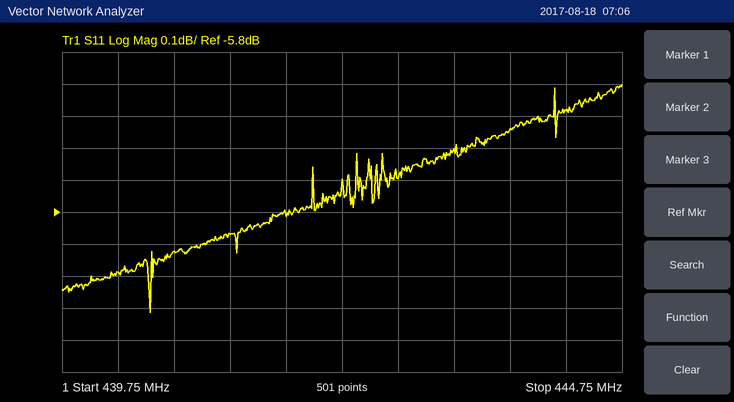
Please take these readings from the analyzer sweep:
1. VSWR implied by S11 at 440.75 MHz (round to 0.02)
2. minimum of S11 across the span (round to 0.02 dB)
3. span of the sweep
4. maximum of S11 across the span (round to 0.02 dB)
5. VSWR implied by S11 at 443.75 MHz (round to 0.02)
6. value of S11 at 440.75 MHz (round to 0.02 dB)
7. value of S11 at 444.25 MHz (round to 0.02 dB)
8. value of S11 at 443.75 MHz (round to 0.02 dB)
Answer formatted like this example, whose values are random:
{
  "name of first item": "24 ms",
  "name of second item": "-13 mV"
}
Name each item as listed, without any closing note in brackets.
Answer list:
{
  "VSWR implied by S11 at 440.75 MHz": "3.04",
  "minimum of S11 across the span": "-6.12 dB",
  "span of the sweep": "5 MHz",
  "maximum of S11 across the span": "-5.40 dB",
  "VSWR implied by S11 at 443.75 MHz": "3.24",
  "value of S11 at 440.75 MHz": "-5.92 dB",
  "value of S11 at 444.25 MHz": "-5.48 dB",
  "value of S11 at 443.75 MHz": "-5.54 dB"
}
